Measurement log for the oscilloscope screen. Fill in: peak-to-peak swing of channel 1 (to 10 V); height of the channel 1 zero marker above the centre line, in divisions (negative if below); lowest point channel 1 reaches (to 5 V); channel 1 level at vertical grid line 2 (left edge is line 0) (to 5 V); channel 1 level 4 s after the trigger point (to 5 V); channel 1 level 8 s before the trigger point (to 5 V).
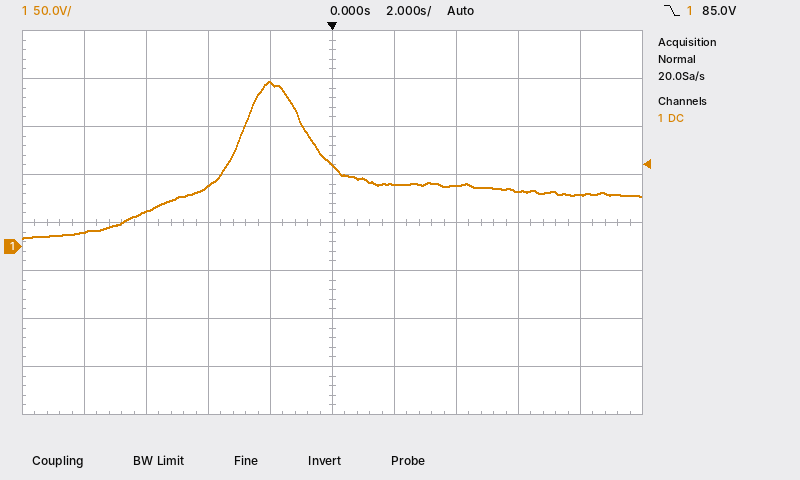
160 V
-0.5 div
10 V
35 V
65 V
15 V
